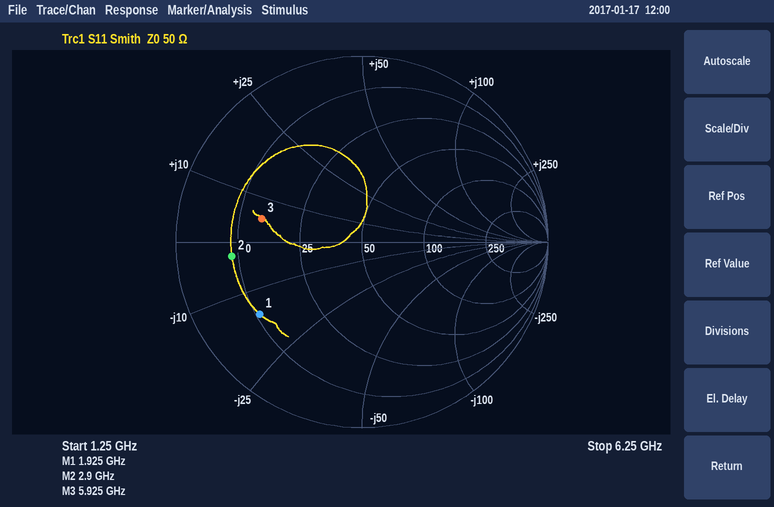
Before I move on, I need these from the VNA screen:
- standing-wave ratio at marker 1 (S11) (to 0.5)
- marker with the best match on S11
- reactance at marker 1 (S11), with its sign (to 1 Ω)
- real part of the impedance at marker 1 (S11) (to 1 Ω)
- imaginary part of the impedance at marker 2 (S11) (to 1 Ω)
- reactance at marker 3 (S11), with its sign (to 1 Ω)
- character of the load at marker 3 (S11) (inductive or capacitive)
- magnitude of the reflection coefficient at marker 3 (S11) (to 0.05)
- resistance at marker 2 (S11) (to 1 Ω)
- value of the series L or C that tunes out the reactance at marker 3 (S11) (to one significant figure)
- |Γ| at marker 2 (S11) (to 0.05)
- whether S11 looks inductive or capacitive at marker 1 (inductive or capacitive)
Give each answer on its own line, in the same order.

5.0
marker 3
-15 Ω
11 Ω
-3 Ω
+5 Ω
inductive
0.55
9 Ω
5 pF
0.70
capacitive
